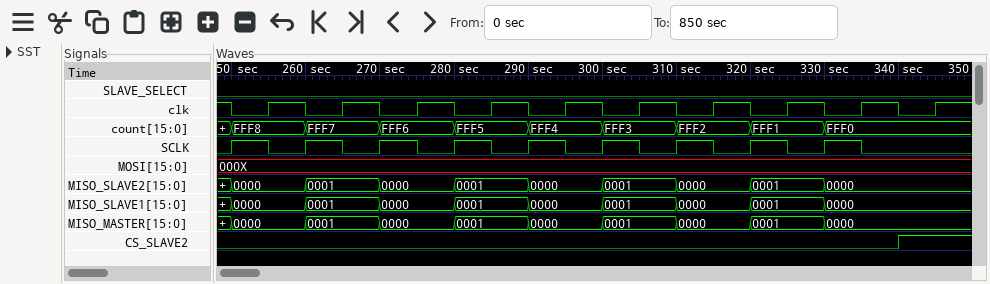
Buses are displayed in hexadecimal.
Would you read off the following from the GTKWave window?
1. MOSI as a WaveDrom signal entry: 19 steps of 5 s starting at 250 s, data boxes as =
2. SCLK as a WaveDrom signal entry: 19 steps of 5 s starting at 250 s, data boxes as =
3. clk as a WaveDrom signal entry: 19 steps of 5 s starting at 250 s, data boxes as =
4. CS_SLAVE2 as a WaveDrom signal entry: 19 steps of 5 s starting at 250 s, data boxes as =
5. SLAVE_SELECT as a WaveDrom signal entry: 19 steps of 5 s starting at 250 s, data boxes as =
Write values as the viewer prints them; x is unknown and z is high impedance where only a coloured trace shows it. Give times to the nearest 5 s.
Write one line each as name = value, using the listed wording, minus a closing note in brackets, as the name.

MOSI as a WaveDrom signal entry: 19 steps of 5 s starting at 250 s, data boxes as = = {name: 'MOSI', wave: '=..................', data: '000X'}
SCLK as a WaveDrom signal entry: 19 steps of 5 s starting at 250 s, data boxes as = = {name: 'SCLK', wave: '101010101010101010.'}
clk as a WaveDrom signal entry: 19 steps of 5 s starting at 250 s, data boxes as = = {name: 'clk', wave: '0101010101010101010'}
CS_SLAVE2 as a WaveDrom signal entry: 19 steps of 5 s starting at 250 s, data boxes as = = {name: 'CS_SLAVE2', wave: '0.................1'}
SLAVE_SELECT as a WaveDrom signal entry: 19 steps of 5 s starting at 250 s, data boxes as = = {name: 'SLAVE_SELECT', wave: '0..................'}
